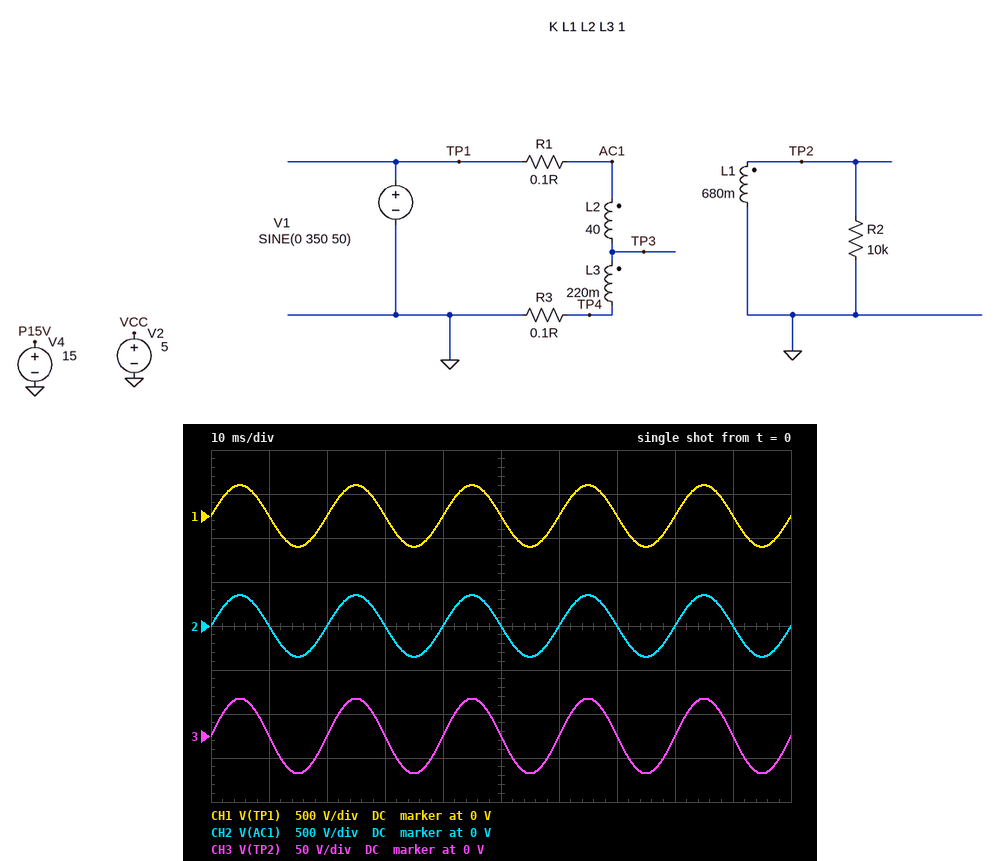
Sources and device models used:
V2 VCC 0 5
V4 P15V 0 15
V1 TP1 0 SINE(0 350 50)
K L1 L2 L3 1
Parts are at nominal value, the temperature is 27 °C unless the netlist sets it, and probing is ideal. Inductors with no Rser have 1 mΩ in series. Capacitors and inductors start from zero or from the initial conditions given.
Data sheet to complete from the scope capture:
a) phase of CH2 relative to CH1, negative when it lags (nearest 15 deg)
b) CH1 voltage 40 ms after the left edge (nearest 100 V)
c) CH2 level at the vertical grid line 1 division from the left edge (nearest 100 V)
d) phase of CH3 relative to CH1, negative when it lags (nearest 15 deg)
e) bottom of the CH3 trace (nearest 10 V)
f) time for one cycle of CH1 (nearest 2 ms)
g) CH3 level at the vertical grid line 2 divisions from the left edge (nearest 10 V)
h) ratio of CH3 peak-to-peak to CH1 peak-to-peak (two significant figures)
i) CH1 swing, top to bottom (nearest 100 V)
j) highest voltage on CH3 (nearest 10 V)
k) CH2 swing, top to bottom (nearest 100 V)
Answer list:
0 deg
0 V
0 V
0 deg
-40 V
20 ms
0 V
0.12
700 V
40 V
700 V
